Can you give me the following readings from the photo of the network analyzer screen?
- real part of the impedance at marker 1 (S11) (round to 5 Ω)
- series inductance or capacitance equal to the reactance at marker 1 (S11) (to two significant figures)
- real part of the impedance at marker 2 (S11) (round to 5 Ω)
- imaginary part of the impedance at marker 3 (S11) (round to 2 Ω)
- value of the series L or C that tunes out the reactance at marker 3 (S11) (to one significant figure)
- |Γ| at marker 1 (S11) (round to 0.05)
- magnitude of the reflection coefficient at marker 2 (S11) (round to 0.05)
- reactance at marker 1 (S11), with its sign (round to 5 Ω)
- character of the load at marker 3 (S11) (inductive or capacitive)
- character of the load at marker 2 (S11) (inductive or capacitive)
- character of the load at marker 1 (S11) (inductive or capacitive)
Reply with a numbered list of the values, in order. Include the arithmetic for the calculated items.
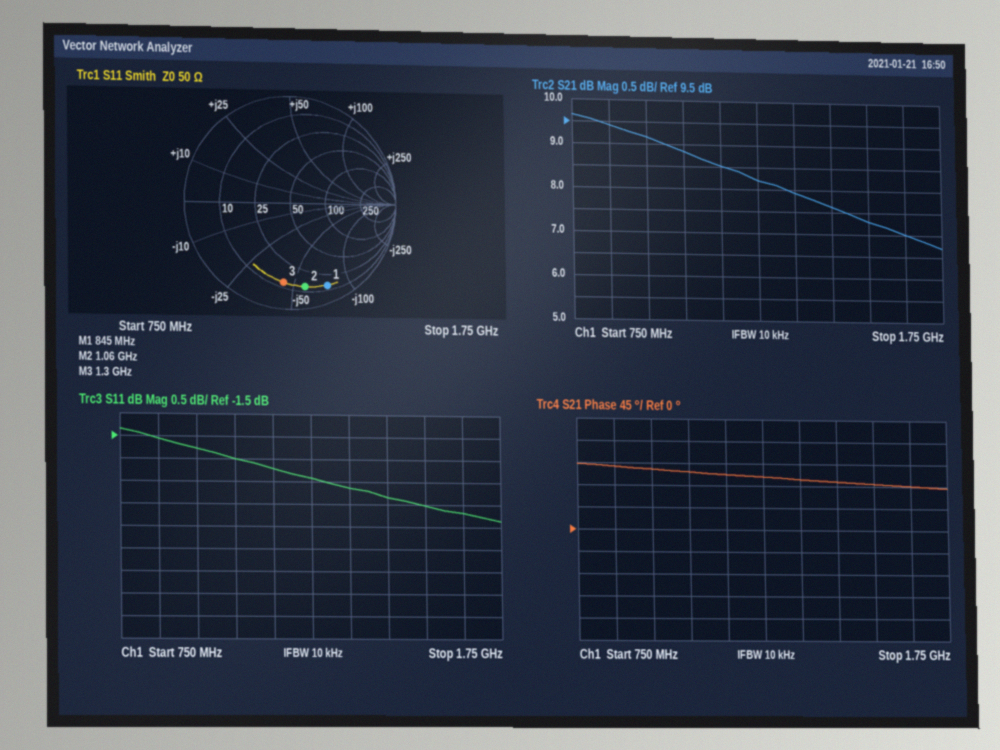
1. 15 Ω
2. C = 1/(2π × 845 MHz × 75 Ω) ≈ 2.5 pF
3. 15 Ω
4. -44 Ω
5. L = 44 Ω/(2π × 1.3 GHz) ≈ 5 nH
6. 0.85
7. 0.80
8. -75 Ω
9. capacitive
10. capacitive
11. capacitive
